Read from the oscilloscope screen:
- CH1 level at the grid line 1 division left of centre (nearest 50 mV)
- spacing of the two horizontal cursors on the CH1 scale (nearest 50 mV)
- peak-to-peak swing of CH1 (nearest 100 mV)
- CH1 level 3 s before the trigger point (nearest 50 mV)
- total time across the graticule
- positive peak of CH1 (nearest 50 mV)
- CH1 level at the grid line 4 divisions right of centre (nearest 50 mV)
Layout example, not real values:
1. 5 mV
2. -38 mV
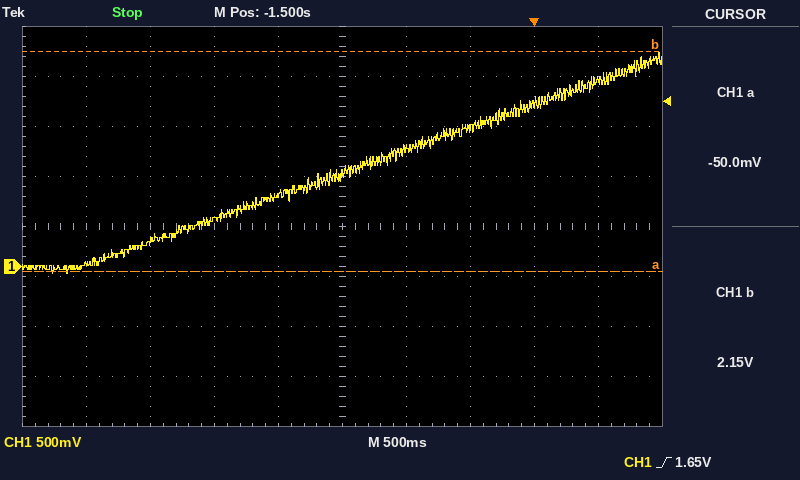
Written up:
1. 750 mV
2. 2.20 V
3. 2.20 V
4. 250 mV
5. 5 s
6. 2.15 V
7. 1.85 V
